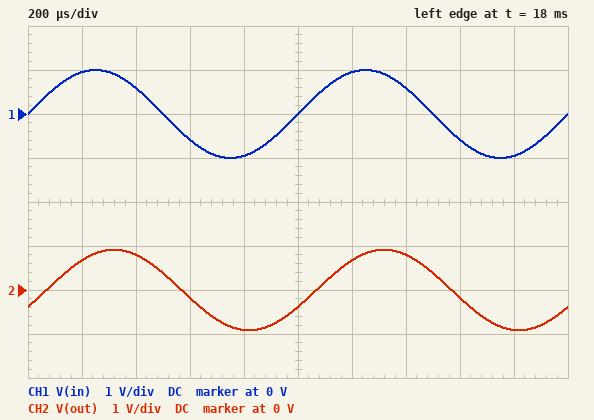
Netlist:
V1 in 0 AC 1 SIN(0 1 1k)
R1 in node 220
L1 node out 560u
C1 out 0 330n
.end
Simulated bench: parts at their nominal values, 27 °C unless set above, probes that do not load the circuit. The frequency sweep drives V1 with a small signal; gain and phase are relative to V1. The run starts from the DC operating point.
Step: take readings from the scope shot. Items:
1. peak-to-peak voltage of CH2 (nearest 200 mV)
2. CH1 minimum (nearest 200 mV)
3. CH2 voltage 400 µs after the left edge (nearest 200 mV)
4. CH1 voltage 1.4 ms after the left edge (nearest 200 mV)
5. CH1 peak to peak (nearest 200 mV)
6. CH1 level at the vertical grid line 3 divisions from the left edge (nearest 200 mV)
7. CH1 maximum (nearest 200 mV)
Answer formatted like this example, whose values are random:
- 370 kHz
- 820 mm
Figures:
- 1.8 V
- -1.0 V
- 800 mV
- 600 mV
- 2.0 V
- -600 mV
- 1.0 V
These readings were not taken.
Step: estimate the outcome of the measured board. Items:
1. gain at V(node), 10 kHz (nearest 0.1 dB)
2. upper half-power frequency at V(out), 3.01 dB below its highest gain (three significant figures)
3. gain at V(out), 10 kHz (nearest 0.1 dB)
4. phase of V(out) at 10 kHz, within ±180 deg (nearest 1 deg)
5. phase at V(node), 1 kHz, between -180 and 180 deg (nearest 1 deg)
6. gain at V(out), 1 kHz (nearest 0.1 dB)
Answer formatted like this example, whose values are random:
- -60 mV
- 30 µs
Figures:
- -24.6 dB
- 2.27 kHz
- -13.2 dB
- -87 deg
- -25 deg
- -0.8 dB
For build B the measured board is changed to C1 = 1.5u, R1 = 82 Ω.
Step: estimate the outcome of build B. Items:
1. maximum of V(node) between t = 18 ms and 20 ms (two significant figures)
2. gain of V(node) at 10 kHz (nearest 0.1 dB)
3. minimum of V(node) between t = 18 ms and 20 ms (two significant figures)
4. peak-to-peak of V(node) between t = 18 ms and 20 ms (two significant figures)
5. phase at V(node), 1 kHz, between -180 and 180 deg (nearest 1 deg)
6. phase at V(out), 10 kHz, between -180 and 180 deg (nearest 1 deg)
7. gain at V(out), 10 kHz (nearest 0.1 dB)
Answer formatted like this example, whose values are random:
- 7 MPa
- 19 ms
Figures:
- 780 mV
- -10.8 dB
- -780 mV
- 1.6 V
- -39 deg
- -107 deg
- -18.1 dB
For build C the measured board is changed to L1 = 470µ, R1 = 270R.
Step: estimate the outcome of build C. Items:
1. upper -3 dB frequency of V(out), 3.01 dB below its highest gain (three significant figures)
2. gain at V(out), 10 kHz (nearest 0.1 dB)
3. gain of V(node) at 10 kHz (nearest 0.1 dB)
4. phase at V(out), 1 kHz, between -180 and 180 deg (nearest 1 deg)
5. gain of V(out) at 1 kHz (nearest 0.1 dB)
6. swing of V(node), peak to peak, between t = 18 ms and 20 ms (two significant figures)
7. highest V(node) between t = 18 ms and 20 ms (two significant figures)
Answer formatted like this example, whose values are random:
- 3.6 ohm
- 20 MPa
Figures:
- 1.82 kHz
- -15.0 dB
- -23.2 dB
- -29 deg
- -1.1 dB
- 1.7 V
- 870 mV
